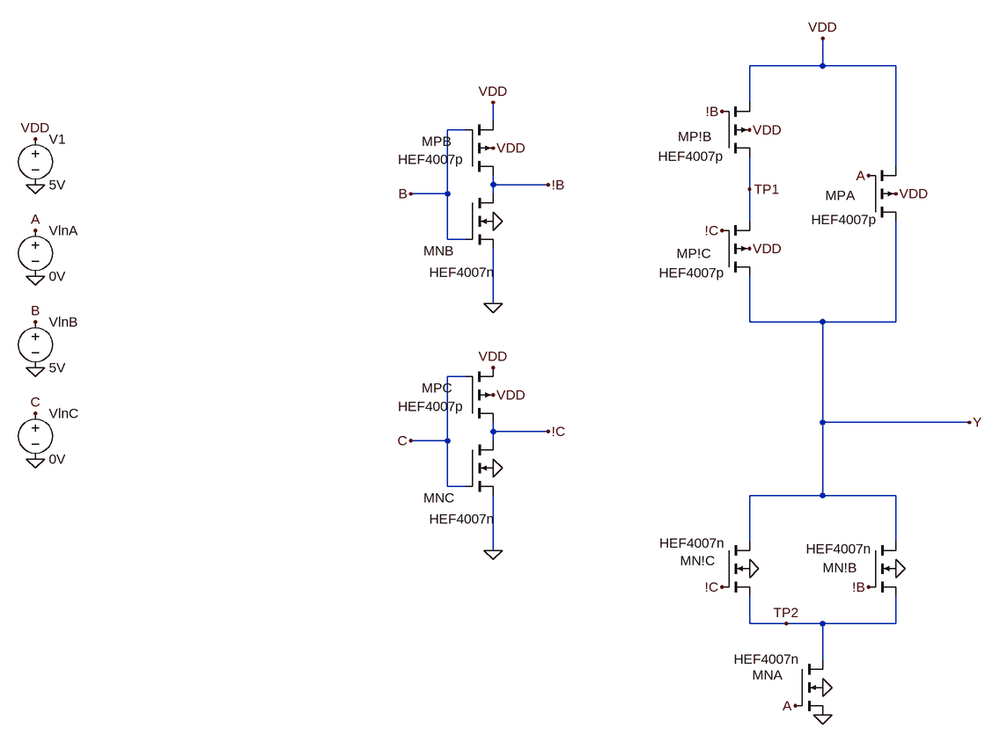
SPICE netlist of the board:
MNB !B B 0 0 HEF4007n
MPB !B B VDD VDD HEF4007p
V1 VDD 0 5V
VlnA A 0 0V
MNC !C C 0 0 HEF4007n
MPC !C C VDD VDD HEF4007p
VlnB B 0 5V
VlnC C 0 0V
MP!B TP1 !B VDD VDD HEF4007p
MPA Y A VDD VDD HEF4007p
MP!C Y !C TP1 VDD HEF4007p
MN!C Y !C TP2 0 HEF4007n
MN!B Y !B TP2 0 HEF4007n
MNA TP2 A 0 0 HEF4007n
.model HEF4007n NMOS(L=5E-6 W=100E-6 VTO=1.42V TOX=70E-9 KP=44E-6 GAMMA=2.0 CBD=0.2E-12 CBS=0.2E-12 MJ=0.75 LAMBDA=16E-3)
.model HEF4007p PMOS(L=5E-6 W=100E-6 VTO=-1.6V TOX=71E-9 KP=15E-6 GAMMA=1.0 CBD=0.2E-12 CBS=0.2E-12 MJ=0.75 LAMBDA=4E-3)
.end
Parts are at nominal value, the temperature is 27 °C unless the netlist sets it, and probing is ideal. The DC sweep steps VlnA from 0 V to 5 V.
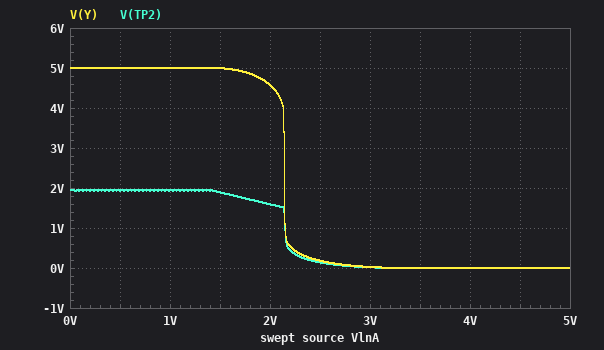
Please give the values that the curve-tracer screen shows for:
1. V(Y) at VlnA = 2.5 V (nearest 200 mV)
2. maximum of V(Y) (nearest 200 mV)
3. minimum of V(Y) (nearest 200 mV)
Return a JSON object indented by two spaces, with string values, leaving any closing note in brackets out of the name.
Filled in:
{
  "V(Y) at VlnA = 2.5 V": "200 mV",
  "maximum of V(Y)": "5.0 V",
  "minimum of V(Y)": "0 V"
}
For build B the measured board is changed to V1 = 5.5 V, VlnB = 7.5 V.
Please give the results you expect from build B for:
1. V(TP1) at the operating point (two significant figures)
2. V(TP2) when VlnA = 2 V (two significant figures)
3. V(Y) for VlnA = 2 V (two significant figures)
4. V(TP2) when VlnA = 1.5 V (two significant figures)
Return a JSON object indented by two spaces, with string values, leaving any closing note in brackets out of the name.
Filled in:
{
  "V(TP1) at the operating point": "5.5 V",
  "V(TP2) when VlnA = 2 V": "1.9 V",
  "V(Y) for VlnA = 2 V": "5.2 V",
  "V(TP2) when VlnA = 1.5 V": "2.2 V"
}
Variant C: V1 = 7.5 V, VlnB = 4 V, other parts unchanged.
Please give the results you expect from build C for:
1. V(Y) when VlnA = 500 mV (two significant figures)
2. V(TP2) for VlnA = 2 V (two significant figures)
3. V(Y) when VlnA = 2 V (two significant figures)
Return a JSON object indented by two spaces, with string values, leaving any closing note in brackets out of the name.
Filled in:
{
  "V(Y) when VlnA = 500 mV": "7.5 V",
  "V(TP2) for VlnA = 2 V": "3.2 V",
  "V(Y) when VlnA = 2 V": "7.4 V"
}
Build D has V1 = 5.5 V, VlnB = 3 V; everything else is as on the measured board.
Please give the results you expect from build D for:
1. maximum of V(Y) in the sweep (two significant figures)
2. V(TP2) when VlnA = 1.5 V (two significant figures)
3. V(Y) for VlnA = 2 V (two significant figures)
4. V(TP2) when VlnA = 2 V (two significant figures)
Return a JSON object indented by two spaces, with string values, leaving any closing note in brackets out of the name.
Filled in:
{
  "maximum of V(Y) in the sweep": "5.5 V",
  "V(TP2) when VlnA = 1.5 V": "2.2 V",
  "V(Y) for VlnA = 2 V": "5.2 V",
  "V(TP2) when VlnA = 2 V": "1.9 V"
}
